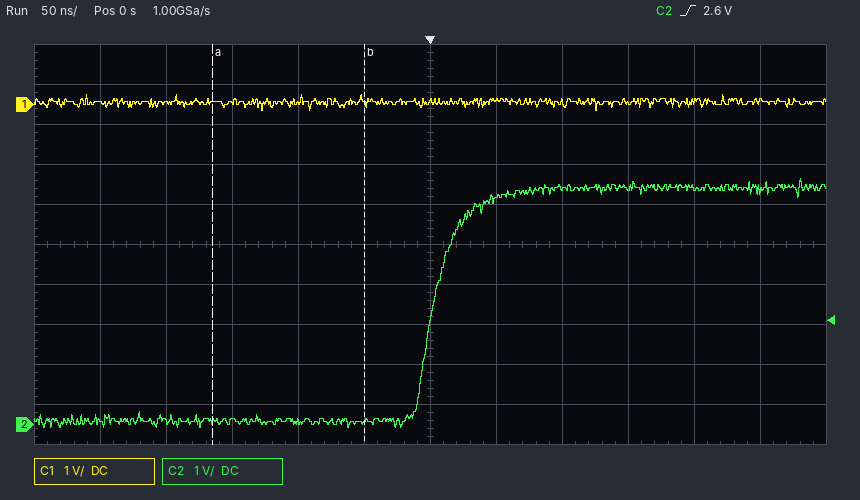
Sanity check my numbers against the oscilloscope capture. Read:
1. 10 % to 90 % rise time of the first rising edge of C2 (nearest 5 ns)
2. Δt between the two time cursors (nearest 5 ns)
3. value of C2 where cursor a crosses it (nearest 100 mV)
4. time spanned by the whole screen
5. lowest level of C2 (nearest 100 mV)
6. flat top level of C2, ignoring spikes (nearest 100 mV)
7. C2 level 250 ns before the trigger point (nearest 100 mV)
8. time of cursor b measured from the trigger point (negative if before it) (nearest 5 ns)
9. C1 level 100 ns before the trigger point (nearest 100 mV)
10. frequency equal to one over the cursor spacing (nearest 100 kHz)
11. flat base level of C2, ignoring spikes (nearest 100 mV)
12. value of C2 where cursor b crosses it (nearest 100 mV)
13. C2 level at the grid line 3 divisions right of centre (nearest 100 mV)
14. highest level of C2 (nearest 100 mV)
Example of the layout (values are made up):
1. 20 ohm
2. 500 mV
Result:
1. 40 ns
2. 115 ns
3. 100 mV
4. 600 ns
5. -100 mV
6. 5.9 V
7. 100 mV
8. -50 ns
9. 100 mV
10. 8.7 MHz
11. 100 mV
12. 100 mV
13. 5.9 V
14. 6.2 V
